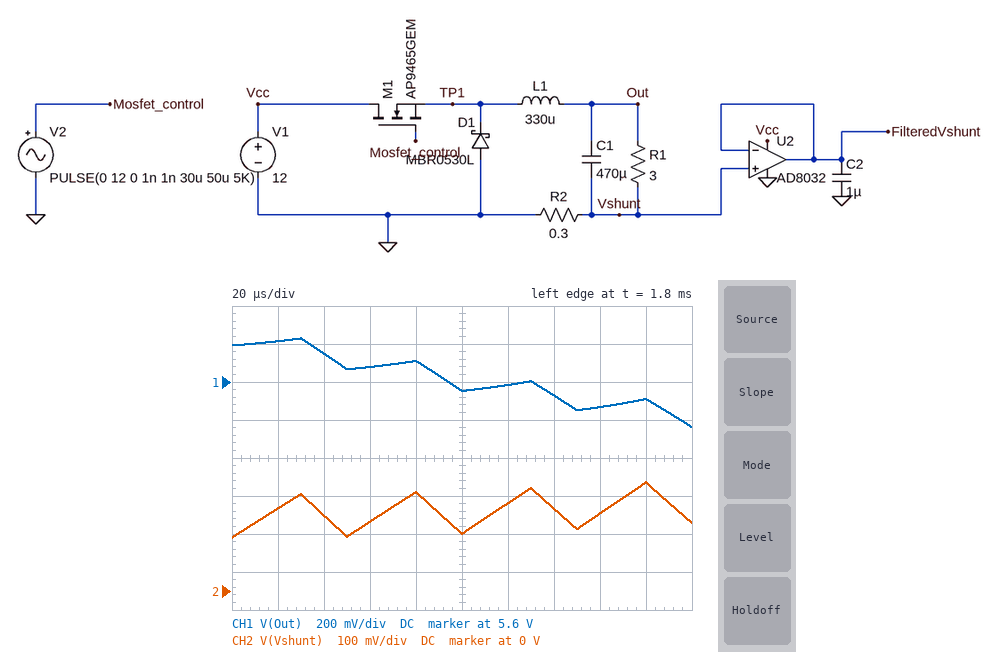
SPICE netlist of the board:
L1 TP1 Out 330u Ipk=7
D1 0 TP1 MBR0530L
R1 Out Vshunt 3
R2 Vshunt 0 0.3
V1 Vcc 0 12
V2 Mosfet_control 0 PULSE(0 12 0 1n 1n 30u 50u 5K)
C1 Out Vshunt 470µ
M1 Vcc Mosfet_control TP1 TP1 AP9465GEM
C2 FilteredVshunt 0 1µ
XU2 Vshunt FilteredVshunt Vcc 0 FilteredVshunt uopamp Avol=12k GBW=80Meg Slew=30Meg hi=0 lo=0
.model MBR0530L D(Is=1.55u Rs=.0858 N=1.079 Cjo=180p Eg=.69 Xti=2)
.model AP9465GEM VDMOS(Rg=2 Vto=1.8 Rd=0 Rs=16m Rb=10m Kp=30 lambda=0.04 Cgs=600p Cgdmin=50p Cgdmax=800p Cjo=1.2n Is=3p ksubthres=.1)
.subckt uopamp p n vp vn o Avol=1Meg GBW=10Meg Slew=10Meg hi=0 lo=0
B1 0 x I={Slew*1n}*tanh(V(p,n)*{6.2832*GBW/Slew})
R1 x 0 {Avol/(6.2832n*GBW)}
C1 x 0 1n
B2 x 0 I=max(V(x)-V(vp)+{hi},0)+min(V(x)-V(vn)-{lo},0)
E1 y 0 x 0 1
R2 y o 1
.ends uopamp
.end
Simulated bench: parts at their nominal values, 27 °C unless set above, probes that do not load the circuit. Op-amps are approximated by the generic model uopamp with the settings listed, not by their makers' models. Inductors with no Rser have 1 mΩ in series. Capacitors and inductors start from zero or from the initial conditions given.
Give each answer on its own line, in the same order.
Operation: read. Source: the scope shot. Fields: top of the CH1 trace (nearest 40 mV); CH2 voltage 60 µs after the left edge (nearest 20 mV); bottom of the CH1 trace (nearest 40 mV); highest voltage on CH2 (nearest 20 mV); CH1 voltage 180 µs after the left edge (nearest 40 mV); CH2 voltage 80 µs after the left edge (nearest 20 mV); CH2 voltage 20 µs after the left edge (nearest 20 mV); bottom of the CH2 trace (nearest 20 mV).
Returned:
5.84 V
180 mV
5.36 V
280 mV
5.52 V
260 mV
220 mV
140 mV
